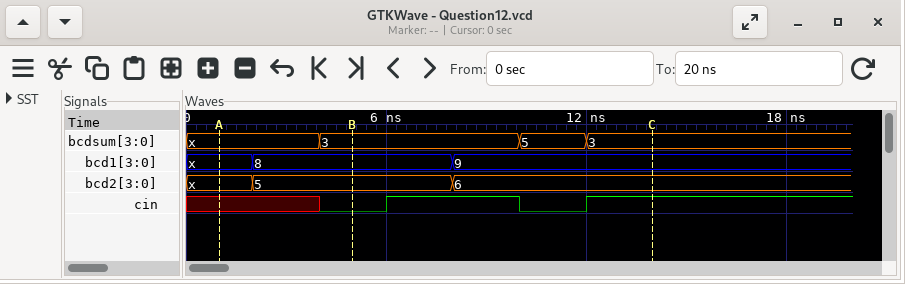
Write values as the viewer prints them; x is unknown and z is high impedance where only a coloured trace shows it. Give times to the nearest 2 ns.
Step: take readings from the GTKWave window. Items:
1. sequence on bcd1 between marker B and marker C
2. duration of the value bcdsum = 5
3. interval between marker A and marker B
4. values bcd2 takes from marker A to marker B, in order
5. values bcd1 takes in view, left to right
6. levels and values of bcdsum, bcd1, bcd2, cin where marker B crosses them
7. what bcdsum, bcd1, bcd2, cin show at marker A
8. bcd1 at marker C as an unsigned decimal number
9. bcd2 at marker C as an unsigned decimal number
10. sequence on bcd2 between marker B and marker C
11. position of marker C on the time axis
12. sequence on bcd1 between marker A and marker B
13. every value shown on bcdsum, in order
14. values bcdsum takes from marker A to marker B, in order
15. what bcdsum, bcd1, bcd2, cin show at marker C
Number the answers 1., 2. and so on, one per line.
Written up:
1. 8, 9
2. 2 ns
3. 4 ns
4. x, 5
5. x, 8, 9
6. bcdsum=3, bcd1=8, bcd2=5, cin=0
7. bcdsum=x, bcd1=x, bcd2=x, cin=x
8. 9
9. 6
10. 5, 6
11. 14 ns
12. x, 8
13. x, 3, 5, 3
14. x, 3
15. bcdsum=3, bcd1=9, bcd2=6, cin=1
